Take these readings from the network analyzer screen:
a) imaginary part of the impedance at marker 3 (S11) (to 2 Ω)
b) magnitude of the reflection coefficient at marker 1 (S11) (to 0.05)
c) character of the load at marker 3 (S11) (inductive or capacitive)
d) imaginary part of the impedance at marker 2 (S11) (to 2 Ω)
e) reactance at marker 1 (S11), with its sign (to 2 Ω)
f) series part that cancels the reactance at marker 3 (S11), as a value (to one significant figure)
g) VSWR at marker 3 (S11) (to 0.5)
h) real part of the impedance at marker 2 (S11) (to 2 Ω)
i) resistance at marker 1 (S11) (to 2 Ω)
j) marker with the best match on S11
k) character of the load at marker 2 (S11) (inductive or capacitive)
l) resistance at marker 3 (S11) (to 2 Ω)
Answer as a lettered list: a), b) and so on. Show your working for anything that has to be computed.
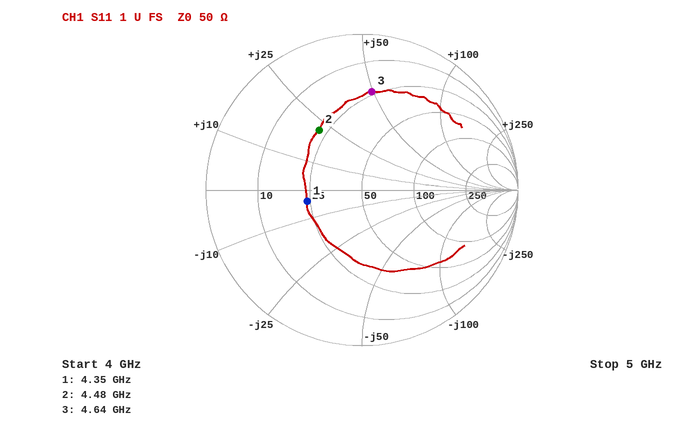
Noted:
a) +50 Ω
b) 0.35
c) inductive
d) +22 Ω
e) -4 Ω
f) C = 1/(2π × 4.64 GHz × 50 Ω) ≈ 686 fF, so 700 fF to one significant figure
g) 4.5
h) 22 Ω
i) 24 Ω
j) marker 1
k) inductive
l) 24 Ω
